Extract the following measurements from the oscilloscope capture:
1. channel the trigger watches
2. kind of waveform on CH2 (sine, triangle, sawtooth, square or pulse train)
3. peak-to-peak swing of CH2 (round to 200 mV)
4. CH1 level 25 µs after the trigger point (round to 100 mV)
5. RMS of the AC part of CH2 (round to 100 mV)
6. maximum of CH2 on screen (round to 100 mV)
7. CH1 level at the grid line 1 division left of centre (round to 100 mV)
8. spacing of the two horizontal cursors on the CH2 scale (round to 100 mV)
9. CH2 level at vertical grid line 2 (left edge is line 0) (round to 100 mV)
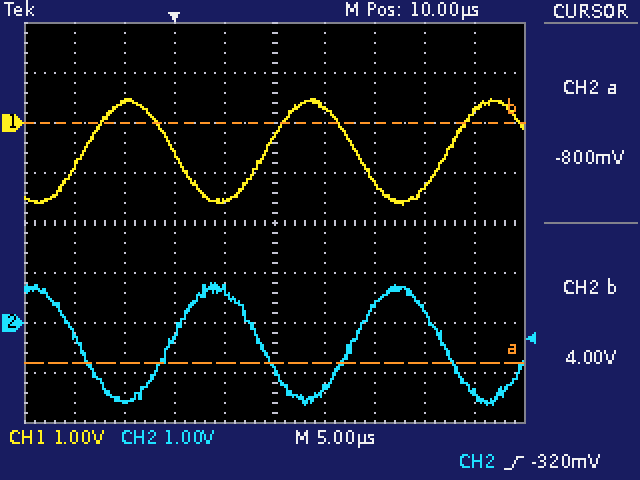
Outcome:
CH2
sine
2.4 V
-1.3 V
800 mV
800 mV
-1.6 V
4.8 V
-1.6 V
